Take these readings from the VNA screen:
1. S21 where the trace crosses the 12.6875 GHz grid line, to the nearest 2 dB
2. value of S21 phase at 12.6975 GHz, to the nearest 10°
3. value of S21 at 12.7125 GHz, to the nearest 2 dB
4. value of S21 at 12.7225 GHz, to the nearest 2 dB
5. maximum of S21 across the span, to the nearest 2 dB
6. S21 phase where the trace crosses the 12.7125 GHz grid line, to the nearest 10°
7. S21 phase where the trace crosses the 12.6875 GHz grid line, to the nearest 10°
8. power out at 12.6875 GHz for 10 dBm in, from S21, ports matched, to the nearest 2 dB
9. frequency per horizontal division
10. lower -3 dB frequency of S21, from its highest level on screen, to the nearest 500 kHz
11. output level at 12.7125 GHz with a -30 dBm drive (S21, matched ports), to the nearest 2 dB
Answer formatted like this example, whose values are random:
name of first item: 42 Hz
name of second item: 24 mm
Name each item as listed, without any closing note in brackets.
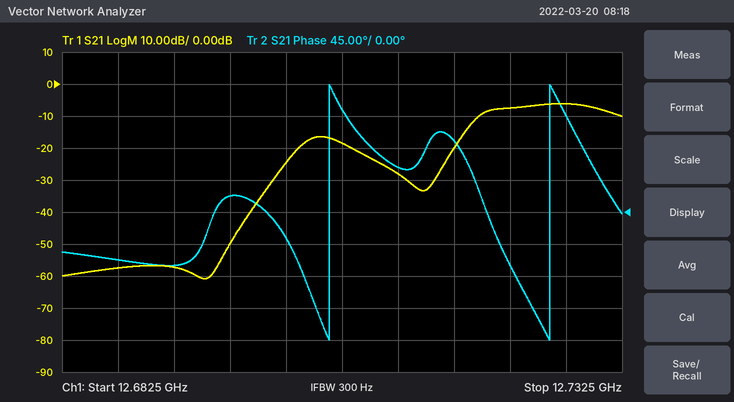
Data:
S21 where the trace crosses the 12.6875 GHz grid line, to the nearest 2 dB: -58 dB
value of S21 phase at 12.6975 GHz, to the nearest 10°: 20°
value of S21 at 12.7125 GHz, to the nearest 2 dB: -28 dB
value of S21 at 12.7225 GHz, to the nearest 2 dB: -8 dB
maximum of S21 across the span, to the nearest 2 dB: -6 dB
S21 phase where the trace crosses the 12.7125 GHz grid line, to the nearest 10°: 60°
S21 phase where the trace crosses the 12.6875 GHz grid line, to the nearest 10°: -70°
power out at 12.6875 GHz for 10 dBm in, from S21, ports matched, to the nearest 2 dB: -48 dBm
frequency per horizontal division: 5 MHz
lower -3 dB frequency of S21, from its highest level on screen, to the nearest 500 kHz: 12.7200 GHz
output level at 12.7125 GHz with a -30 dBm drive (S21, matched ports), to the nearest 2 dB: -58 dBm
